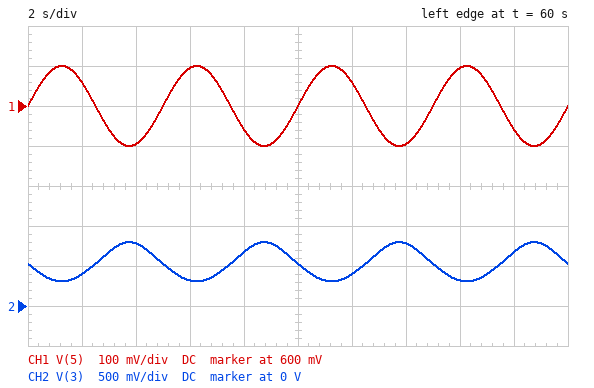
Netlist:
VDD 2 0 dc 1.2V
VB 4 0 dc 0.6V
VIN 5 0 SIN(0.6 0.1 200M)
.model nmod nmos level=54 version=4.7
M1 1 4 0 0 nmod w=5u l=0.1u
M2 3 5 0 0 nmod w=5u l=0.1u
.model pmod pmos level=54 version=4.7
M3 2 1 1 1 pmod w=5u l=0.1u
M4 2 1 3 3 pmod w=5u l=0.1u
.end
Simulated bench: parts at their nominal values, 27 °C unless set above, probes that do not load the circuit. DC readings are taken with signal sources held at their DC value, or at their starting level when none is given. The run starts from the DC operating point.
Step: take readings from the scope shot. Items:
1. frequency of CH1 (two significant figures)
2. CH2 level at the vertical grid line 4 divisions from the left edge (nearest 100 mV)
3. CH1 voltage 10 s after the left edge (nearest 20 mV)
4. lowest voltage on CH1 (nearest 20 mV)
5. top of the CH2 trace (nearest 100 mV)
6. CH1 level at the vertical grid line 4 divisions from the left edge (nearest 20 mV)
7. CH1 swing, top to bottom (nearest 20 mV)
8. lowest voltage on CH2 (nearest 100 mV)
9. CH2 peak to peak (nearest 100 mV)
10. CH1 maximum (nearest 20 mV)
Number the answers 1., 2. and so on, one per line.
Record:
1. 200 mHz
2. 700 mV
3. 600 mV
4. 500 mV
5. 800 mV
6. 540 mV
7. 200 mV
8. 300 mV
9. 500 mV
10. 700 mV
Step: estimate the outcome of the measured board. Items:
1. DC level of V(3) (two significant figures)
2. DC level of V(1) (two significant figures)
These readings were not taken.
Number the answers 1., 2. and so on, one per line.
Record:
1. 530 mV
2. 530 mV
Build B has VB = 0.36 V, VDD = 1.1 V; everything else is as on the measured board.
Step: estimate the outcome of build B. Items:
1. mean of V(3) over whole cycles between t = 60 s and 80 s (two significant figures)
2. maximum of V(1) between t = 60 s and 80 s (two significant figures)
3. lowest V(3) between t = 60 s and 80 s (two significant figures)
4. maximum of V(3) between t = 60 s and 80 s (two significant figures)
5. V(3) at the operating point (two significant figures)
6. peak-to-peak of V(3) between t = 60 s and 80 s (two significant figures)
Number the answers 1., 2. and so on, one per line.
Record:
1. 92 mV
2. 700 mV
3. 49 mV
4. 190 mV
5. 72 mV
6. 140 mV
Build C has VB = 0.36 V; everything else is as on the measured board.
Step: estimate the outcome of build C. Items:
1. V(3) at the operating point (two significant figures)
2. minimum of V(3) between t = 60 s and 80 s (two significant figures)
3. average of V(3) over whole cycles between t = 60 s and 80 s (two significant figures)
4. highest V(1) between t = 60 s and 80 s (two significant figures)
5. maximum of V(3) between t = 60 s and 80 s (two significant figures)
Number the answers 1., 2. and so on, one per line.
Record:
1. 84 mV
2. 56 mV
3. 110 mV
4. 790 mV
5. 230 mV
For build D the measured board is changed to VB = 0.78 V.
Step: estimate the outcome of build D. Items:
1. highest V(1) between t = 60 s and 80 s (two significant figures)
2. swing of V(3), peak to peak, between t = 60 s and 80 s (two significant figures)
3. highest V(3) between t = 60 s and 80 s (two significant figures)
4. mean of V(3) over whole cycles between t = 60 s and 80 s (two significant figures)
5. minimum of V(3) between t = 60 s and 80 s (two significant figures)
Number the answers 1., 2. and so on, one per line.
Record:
1. 380 mV
2. 440 mV
3. 970 mV
4. 740 mV
5. 530 mV
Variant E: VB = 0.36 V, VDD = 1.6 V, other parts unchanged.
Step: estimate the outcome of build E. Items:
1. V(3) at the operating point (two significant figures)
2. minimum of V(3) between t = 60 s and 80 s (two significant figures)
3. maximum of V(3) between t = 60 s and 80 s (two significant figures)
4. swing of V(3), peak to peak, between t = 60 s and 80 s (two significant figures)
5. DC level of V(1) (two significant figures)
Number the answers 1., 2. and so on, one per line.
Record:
1. 160 mV
2. 92 mV
3. 450 mV
4. 360 mV
5. 1.2 V
